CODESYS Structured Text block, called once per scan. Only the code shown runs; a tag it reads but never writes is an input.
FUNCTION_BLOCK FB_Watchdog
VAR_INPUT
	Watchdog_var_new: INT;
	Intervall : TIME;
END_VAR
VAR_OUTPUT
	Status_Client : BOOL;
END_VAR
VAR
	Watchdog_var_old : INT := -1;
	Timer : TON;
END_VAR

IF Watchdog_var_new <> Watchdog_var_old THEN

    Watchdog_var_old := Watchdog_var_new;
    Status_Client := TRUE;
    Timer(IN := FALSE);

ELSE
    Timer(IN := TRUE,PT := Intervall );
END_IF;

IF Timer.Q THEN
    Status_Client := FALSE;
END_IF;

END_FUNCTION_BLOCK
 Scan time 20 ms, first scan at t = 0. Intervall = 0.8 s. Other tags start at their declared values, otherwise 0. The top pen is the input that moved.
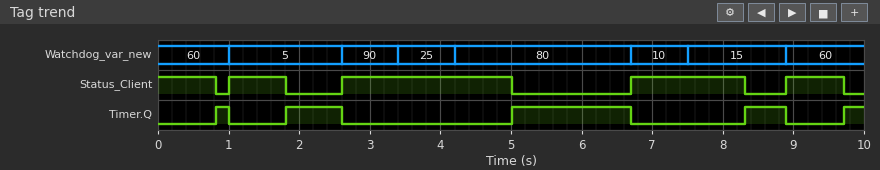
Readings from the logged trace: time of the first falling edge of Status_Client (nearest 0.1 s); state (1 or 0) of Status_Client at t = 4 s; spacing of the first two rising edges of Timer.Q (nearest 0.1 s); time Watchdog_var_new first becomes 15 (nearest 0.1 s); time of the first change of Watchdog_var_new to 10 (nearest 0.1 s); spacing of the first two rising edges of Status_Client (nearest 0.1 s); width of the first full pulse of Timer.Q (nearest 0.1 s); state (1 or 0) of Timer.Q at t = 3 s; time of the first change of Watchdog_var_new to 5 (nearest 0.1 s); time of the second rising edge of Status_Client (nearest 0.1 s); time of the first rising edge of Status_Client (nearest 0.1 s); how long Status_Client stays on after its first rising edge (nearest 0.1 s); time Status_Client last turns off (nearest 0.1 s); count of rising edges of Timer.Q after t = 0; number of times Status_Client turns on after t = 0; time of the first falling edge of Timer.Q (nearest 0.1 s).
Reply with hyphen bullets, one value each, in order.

- 0.8 s
- 1
- 1.0 s
- 7.5 s
- 6.7 s
- 1.6 s
- 0.2 s
- 0
- 1.0 s
- 2.6 s
- 1.0 s
- 0.8 s
- 9.7 s
- 5
- 4
- 1.0 s
